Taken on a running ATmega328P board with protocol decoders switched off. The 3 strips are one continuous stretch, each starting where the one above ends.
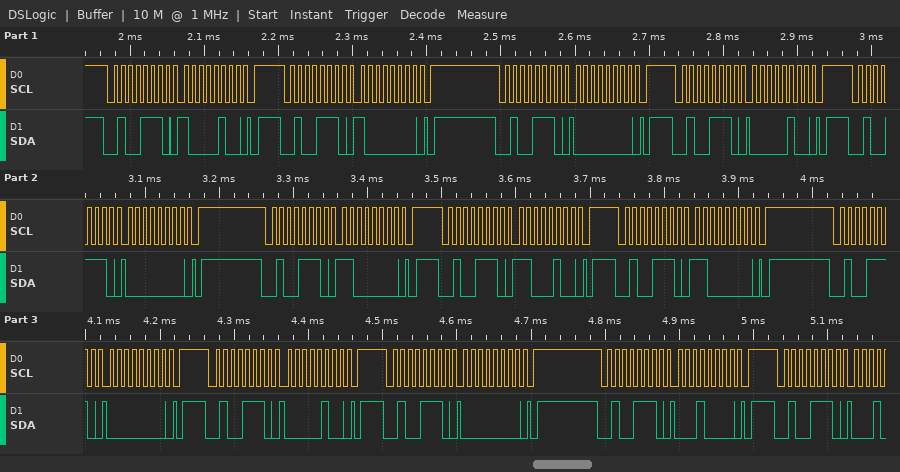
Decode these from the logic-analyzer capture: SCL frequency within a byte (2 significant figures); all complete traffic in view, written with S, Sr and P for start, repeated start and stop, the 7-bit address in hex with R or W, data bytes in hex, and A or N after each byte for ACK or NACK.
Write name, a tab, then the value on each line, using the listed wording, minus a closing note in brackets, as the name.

SCL frequency within a byte	100 kHz
all complete traffic in view, written with S, Sr and P for start, repeated start and stop, the 7-bit address in hex with R or W, data bytes in hex, and A or N after each byte for ACK or NACK	S 27W A 84 A P S 27W A 80 A P S 27W A 00 A P S 27W A 04 A P S 27W A 00 A P S 27W A C0 A P S 27W A C4 A P S 27W A C0 A P S 27W A 00 A P S 27W A 04 A P S 27W A 00 A P S 27W A 10 A P S 27W A
